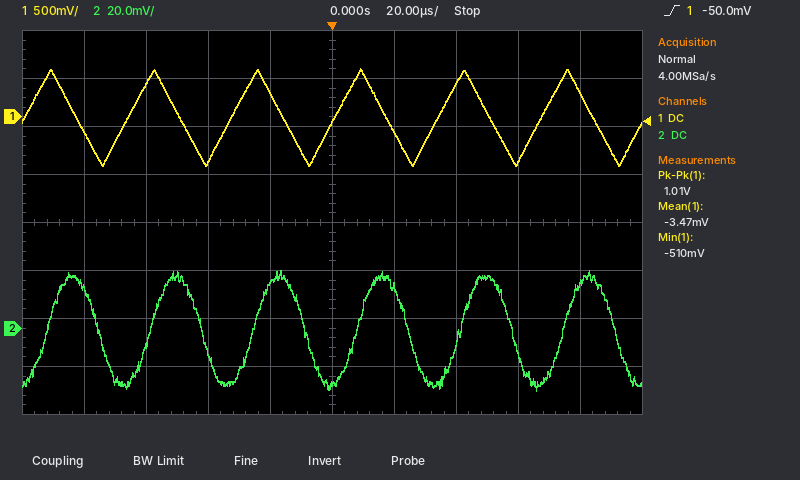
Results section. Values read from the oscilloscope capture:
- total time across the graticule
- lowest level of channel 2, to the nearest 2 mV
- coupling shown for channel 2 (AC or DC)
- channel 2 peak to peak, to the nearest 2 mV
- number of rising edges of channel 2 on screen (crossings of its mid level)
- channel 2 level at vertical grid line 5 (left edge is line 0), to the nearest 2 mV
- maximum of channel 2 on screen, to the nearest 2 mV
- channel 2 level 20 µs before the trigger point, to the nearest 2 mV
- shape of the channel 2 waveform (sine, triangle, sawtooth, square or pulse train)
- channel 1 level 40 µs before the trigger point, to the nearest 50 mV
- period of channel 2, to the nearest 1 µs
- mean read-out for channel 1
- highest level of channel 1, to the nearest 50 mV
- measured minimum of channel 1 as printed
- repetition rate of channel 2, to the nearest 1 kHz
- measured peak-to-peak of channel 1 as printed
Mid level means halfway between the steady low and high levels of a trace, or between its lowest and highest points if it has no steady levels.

200 µs
-26 mV
DC
50 mV
6
-24 mV
24 mV
18 mV
sine
-450 mV
33 µs
-3.47 mV
500 mV
-510 mV
30 kHz
1.01 V
